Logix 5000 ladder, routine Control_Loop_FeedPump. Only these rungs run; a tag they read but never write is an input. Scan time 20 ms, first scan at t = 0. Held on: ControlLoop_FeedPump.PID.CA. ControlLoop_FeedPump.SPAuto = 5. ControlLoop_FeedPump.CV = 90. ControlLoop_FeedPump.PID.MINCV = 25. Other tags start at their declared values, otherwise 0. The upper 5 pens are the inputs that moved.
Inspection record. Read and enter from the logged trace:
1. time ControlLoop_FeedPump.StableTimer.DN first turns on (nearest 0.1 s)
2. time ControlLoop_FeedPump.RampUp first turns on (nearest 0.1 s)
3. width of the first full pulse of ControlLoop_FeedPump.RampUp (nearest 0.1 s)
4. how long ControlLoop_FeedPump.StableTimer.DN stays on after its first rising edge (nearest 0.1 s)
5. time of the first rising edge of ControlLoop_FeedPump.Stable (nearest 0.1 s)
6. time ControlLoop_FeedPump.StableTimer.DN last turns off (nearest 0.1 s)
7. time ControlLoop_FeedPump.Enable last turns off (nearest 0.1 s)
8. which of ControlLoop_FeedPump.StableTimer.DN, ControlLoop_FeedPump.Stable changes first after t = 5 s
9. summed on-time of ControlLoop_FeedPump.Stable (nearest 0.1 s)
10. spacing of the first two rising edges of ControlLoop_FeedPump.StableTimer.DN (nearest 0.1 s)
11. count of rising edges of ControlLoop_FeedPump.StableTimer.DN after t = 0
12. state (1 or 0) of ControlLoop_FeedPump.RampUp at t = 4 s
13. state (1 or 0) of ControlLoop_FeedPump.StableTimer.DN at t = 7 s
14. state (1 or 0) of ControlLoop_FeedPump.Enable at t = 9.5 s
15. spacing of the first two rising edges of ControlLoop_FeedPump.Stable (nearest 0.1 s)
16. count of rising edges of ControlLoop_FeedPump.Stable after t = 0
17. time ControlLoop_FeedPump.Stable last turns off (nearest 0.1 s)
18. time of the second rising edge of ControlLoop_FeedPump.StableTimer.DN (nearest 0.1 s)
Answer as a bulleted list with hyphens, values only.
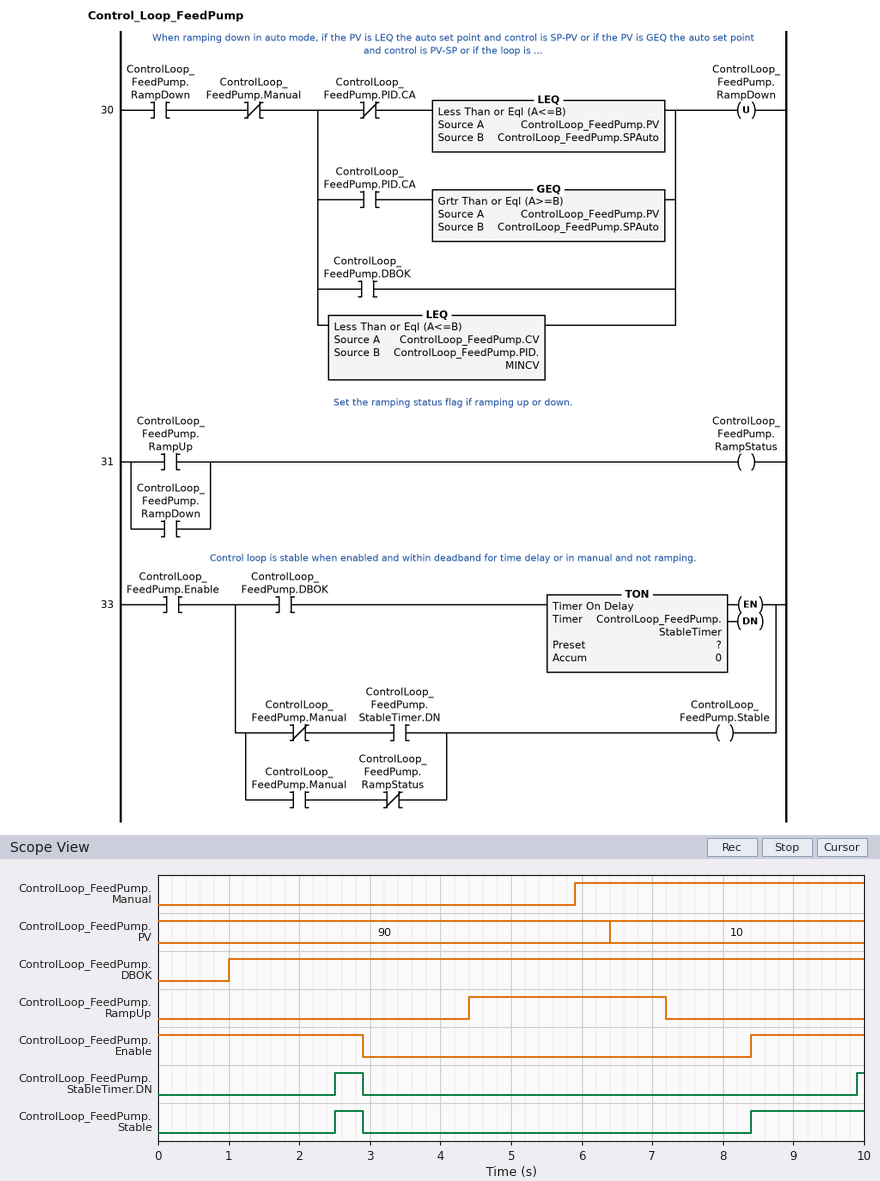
- 2.5 s
- 4.4 s
- 2.8 s
- 0.4 s
- 2.5 s
- 2.9 s
- 2.9 s
- ControlLoop_FeedPump.Stable
- 2.0 s
- 7.4 s
- 2
- 0
- 0
- 1
- 5.9 s
- 2
- 2.9 s
- 9.9 s
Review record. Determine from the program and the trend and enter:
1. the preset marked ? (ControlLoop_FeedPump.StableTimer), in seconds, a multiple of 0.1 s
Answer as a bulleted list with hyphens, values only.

- 1.5 s
